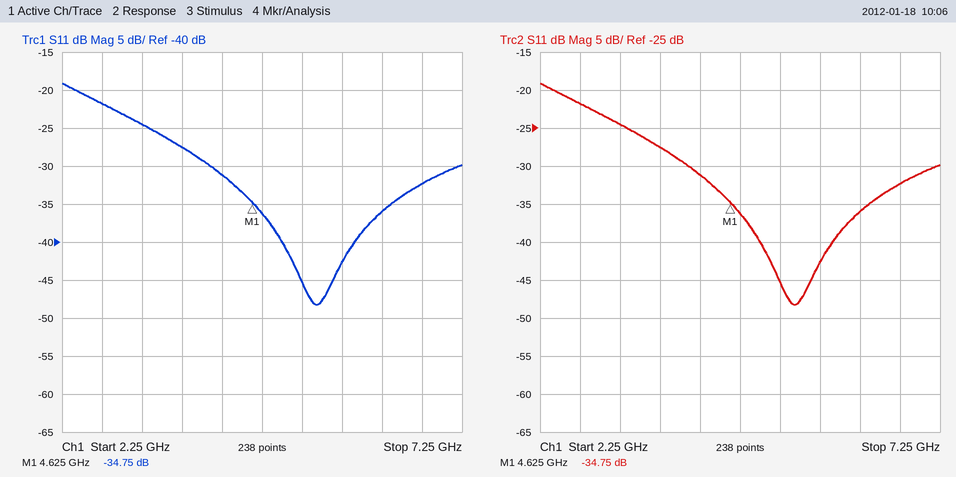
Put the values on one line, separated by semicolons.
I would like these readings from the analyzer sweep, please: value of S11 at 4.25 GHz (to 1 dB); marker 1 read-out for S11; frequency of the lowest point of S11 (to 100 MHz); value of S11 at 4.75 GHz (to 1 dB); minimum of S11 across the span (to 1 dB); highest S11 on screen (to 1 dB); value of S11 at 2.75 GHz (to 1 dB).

-31 dB; -34.75 dB; 5.4 GHz; -36 dB; -48 dB; -19 dB; -22 dB
